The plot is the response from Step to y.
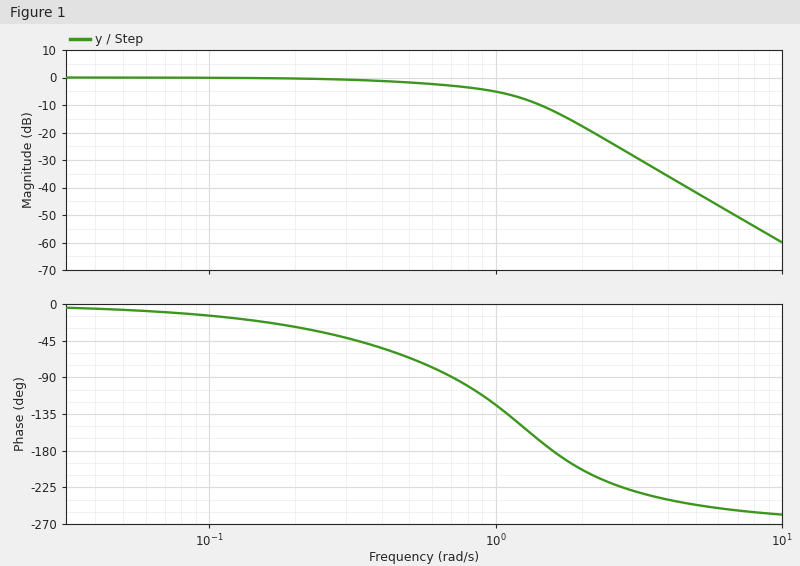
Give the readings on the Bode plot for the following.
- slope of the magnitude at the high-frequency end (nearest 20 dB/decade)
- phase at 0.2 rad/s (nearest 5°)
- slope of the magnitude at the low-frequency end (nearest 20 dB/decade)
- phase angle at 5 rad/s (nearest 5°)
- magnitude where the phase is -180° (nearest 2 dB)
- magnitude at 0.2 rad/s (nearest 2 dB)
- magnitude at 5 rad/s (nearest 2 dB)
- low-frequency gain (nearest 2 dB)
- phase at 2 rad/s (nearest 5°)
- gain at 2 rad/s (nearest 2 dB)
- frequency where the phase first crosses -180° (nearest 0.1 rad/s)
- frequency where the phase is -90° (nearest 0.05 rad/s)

-60 dB/decade
-30°
0 dB/decade
-245°
-12 dB
0 dB
-42 dB
0 dB
-205°
-18 dB
1.6 rad/s
0.70 rad/s
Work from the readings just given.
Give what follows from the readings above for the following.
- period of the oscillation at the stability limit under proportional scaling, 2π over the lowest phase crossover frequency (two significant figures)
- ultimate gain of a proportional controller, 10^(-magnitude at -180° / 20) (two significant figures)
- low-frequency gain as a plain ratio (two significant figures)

3.9 s
4.0
1.0
